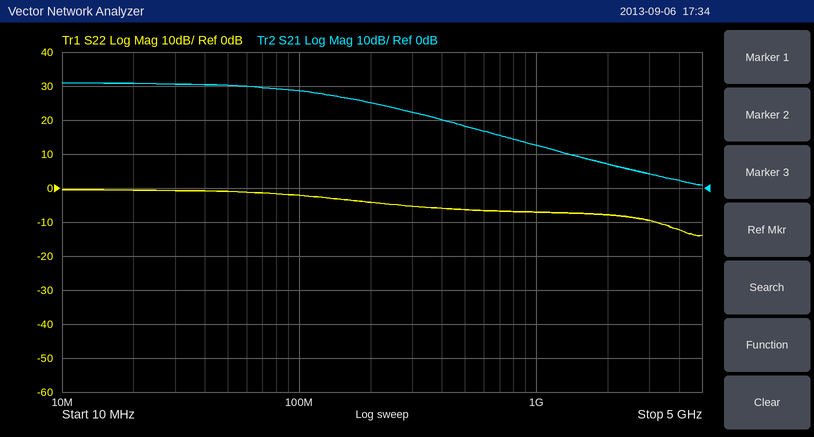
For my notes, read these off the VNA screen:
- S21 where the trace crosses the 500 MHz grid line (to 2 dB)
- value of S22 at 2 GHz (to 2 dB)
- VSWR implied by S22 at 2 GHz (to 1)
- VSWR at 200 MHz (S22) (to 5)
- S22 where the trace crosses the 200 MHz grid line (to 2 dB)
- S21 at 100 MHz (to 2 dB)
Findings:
18 dB
-8 dB
2
5
-4 dB
28 dB
